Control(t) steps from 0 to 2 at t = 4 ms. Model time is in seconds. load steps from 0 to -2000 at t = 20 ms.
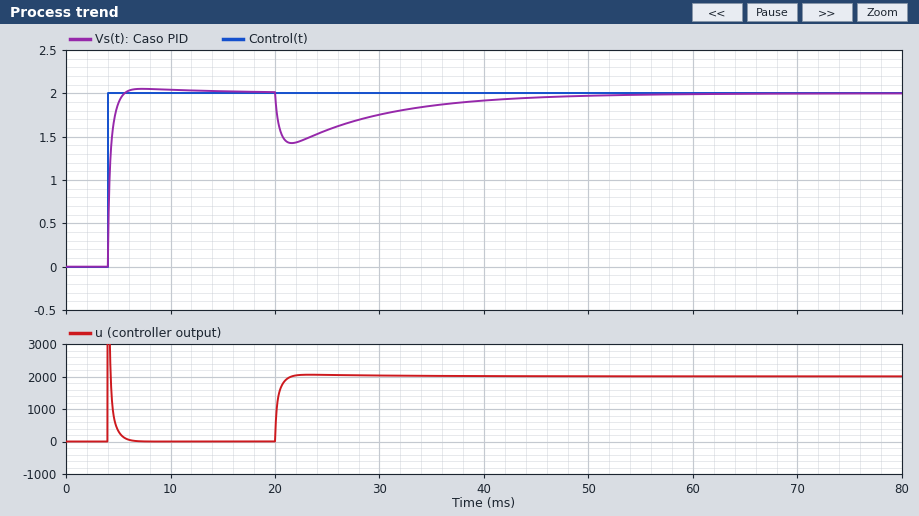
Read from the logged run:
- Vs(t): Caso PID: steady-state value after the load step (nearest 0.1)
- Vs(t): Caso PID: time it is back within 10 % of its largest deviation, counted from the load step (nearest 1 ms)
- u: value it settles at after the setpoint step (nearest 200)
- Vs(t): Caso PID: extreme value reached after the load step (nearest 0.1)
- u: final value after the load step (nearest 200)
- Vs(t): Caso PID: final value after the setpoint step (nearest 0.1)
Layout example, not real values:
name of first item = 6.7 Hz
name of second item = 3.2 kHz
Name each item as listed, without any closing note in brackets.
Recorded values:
Vs(t): Caso PID: steady-state value after the load step = 2.0
Vs(t): Caso PID: time it is back within 10 % of its largest deviation, counted from the load step = 23 ms
u: value it settles at after the setpoint step = 0
Vs(t): Caso PID: extreme value reached after the load step = 1.4
u: final value after the load step = 2000
Vs(t): Caso PID: final value after the setpoint step = 2.0
